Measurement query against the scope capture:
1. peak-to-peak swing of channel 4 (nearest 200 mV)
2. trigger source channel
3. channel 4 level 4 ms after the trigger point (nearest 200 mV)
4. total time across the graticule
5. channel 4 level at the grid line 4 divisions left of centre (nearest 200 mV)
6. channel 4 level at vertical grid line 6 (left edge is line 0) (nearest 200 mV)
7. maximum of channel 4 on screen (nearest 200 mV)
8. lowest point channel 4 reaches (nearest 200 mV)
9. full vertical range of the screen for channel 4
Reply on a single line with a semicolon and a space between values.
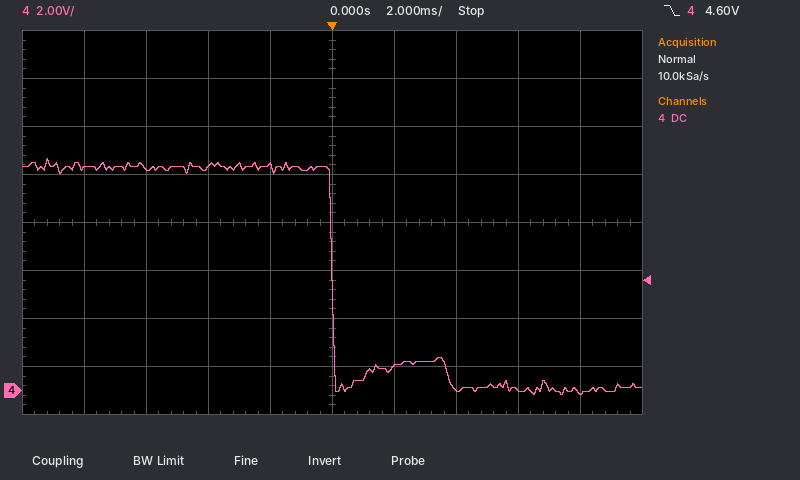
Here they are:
9.8 V; channel 4; 0.0 V; 20 ms; 9.2 V; 1.0 V; 9.6 V; -200 mV; 16 V
